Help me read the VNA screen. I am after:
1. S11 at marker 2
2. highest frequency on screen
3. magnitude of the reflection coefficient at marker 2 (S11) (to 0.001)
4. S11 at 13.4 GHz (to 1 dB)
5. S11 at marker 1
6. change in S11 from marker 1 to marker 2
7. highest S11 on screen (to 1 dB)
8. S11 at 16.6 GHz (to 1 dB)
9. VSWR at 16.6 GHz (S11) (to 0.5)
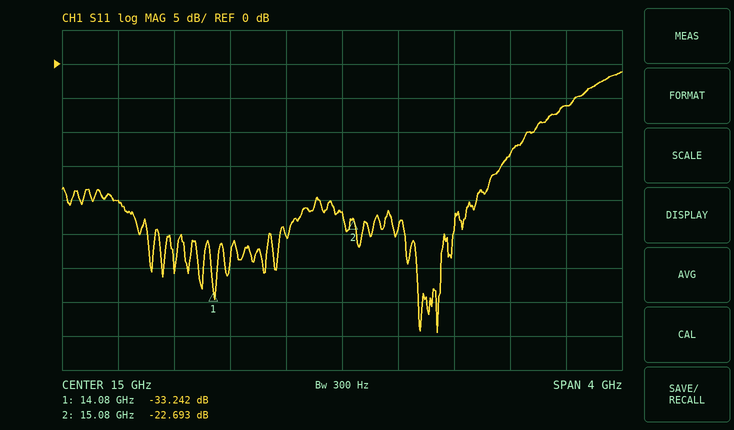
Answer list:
-22.693 dB
17 GHz
0.073
-20 dB
-33.242 dB
10.549 dB
-1 dB
-6 dB
3.0
